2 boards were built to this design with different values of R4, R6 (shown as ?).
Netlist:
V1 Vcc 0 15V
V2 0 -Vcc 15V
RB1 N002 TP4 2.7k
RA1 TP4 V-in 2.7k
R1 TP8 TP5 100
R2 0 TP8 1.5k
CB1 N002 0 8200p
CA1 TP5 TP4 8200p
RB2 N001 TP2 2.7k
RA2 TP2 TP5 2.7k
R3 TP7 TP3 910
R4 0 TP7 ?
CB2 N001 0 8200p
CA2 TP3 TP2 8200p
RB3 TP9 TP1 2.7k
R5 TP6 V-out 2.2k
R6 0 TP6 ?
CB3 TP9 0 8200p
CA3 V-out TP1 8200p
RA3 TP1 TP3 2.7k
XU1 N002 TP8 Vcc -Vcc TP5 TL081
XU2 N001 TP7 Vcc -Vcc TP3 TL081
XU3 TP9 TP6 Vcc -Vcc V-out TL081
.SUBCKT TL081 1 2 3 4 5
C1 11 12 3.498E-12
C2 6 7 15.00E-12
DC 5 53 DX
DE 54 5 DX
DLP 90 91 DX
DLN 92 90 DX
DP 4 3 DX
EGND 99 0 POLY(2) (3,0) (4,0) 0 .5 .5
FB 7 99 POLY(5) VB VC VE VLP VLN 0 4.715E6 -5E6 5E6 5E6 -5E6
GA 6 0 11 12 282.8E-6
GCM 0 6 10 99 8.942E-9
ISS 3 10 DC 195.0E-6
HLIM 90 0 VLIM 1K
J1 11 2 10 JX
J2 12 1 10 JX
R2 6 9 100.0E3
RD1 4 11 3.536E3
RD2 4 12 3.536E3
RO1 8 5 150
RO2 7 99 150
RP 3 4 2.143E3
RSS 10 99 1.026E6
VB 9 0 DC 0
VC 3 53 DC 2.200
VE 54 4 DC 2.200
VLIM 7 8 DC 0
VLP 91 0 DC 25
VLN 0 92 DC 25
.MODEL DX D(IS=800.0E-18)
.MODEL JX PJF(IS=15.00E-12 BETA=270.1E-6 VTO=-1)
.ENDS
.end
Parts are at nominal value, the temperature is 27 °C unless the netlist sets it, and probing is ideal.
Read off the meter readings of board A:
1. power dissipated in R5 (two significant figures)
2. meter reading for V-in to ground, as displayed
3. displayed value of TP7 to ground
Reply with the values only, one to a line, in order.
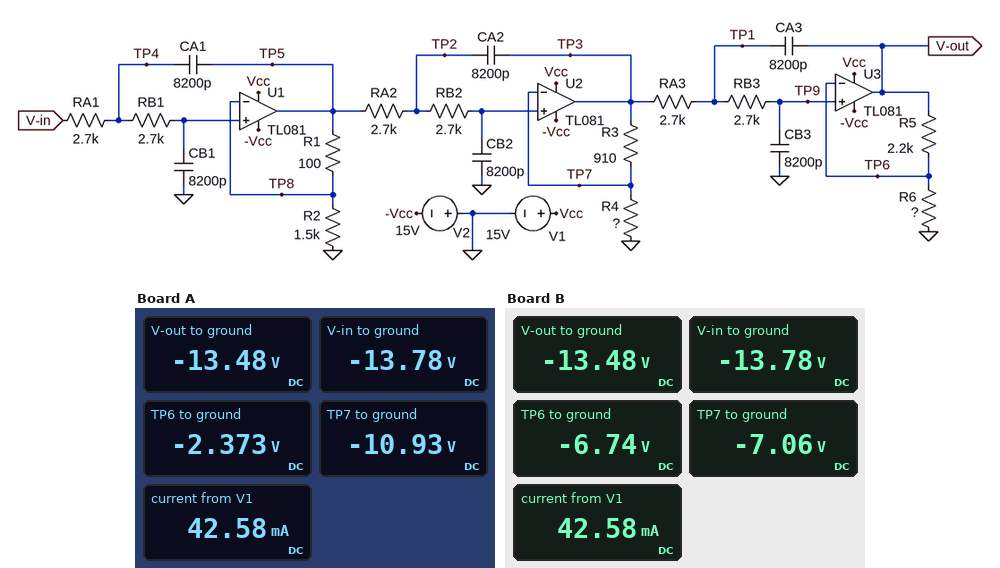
56 mW
-13.78 V
-10.93 V
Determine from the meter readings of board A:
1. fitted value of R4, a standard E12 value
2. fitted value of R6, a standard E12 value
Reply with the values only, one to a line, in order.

3.9 kΩ
470 Ω
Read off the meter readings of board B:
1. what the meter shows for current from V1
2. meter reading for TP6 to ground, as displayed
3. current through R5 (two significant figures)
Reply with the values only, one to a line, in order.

42.58 mA
-6.74 V
3.1 mA
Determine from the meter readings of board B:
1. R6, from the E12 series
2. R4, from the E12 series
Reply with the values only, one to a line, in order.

2.2 kΩ
1 kΩ
